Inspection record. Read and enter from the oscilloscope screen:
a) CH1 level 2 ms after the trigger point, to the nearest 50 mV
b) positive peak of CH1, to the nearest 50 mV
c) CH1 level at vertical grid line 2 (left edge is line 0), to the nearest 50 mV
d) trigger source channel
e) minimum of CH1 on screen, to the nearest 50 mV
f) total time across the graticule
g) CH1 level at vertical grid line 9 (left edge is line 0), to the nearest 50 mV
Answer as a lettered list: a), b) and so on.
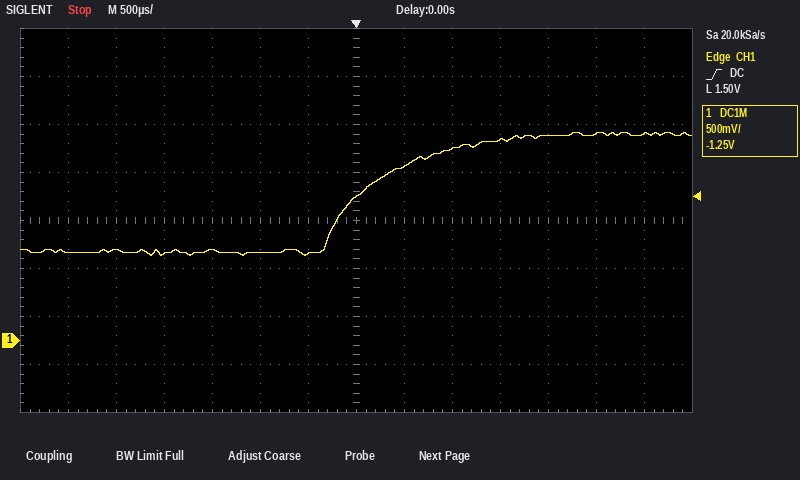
a) 2.15 V
b) 2.15 V
c) 950 mV
d) CH1
e) 900 mV
f) 7 ms
g) 2.00 V
